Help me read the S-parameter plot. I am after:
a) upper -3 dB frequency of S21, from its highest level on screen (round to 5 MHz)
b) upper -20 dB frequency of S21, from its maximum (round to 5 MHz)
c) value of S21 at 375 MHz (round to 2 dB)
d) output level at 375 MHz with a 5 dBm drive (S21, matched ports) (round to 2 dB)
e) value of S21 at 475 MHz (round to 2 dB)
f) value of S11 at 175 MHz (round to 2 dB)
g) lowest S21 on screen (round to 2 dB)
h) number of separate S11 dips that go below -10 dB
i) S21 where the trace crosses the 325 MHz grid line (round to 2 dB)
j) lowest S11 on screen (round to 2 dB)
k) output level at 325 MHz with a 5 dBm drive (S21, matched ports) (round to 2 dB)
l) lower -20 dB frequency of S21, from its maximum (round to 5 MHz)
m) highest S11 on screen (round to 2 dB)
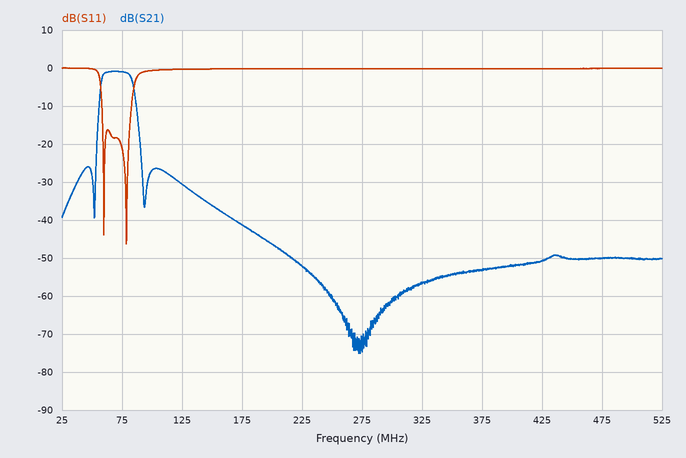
85 MHz
90 MHz
-54 dB
-48 dBm
-50 dB
0 dB
-76 dB
2
-56 dB
-46 dB
-52 dBm
55 MHz
0 dB
